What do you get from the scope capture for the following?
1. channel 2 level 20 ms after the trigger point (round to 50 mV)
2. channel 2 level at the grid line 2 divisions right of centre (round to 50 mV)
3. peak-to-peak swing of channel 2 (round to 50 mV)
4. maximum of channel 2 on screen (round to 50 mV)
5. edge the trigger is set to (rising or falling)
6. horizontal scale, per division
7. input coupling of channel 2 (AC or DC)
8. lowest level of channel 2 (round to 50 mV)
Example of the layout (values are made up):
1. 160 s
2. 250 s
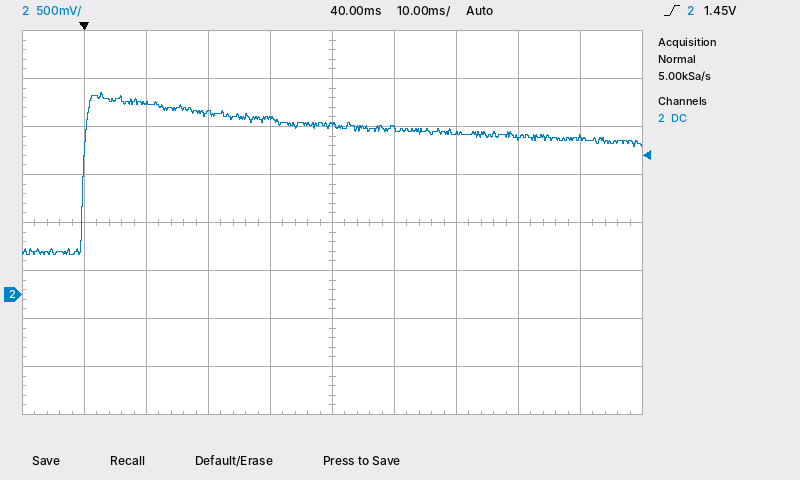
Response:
1. 1.90 V
2. 1.70 V
3. 1.70 V
4. 2.10 V
5. rising
6. 10 ms
7. DC
8. 400 mV
